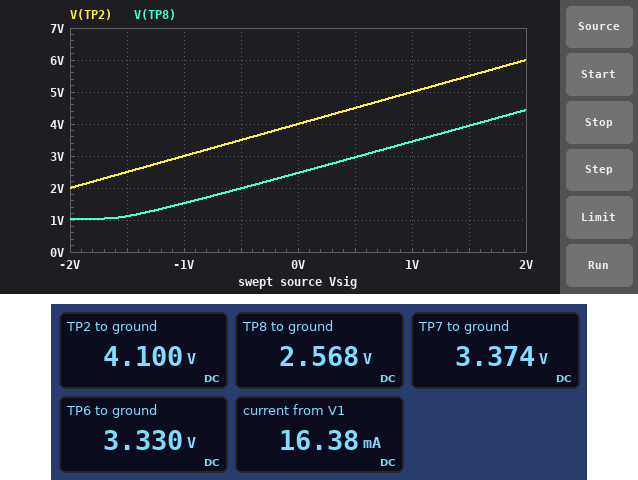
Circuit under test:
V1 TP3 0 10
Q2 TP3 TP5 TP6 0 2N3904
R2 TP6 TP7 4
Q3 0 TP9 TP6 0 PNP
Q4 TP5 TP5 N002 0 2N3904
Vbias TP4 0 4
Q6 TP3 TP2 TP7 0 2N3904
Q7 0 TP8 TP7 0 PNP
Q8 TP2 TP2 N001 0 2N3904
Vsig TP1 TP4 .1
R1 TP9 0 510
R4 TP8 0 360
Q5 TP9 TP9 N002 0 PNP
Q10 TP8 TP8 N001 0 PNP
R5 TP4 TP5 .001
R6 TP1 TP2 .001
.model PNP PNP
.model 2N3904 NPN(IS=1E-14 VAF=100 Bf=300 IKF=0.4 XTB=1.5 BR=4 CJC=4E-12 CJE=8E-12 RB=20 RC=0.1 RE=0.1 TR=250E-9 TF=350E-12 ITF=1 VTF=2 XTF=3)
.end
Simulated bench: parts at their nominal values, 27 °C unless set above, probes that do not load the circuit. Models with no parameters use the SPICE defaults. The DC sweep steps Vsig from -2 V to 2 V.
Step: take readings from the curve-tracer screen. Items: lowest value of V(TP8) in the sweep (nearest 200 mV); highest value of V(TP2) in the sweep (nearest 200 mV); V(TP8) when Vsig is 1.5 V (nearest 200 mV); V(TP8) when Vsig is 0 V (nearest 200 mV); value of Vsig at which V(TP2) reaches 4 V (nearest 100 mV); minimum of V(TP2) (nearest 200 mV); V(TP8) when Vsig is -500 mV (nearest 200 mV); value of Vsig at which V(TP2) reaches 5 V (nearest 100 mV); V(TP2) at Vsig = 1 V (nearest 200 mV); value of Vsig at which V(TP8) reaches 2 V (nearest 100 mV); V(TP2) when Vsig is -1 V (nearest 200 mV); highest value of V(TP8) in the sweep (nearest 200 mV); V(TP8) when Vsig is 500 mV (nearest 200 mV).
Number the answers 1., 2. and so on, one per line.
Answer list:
1. 1.0 V
2. 6.0 V
3. 4.0 V
4. 2.4 V
5. 0 V
6. 2.0 V
7. 2.0 V
8. 1.0 V
9. 5.0 V
10. -500 mV
11. 3.0 V
12. 4.4 V
13. 3.0 V
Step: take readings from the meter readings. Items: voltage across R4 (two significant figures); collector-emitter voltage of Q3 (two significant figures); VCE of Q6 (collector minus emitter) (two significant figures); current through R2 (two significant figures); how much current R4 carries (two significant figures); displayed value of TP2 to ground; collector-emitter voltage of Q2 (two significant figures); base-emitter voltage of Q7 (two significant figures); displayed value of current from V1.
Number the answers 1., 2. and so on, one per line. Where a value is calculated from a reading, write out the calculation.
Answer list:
1. 2.568 V = 2.6 V
2. 0 V - 3.33 V = -3.3 V
3. 10 V - 3.374 V = 6.6 V
4. (3.374 V - 3.33 V) / 4 Ω = 11 mA
5. (2.568 V) / 360 Ω = 7.1 mA
6. 4.100 V
7. 10 V - 3.33 V = 6.7 V
8. 2.568 V - 3.374 V = -810 mV
9. 16.38 mA
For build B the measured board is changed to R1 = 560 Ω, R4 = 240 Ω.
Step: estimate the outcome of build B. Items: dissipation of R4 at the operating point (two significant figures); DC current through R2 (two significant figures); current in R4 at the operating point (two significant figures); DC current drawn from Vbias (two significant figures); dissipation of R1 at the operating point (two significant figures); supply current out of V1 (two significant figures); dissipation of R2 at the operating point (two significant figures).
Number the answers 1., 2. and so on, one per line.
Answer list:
1. 27 mW
2. 9.7 mA
3. 11 mA
4. 15 mA
5. 11 mW
6. 18 mA
7. 380 µW
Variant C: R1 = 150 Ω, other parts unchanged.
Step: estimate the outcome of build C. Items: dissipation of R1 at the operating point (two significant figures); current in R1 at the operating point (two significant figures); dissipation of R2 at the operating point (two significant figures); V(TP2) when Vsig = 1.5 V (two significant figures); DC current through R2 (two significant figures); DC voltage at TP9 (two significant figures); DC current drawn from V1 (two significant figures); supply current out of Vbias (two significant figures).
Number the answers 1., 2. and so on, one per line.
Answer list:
1. 39 mW
2. 16 mA
3. 1.5 mW
4. 5.5 V
5. 19 mA
6. 2.4 V
7. 31 mA
8. 23 mA
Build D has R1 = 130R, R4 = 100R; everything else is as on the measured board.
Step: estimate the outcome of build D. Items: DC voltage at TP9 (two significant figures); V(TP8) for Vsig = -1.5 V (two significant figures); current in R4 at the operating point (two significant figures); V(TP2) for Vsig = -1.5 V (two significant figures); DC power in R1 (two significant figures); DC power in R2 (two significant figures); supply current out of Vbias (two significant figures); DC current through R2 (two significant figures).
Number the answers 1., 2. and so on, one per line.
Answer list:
1. 2.4 V
2. 970 mV
3. 25 mA
4. 2.5 V
5. 45 mW
6. 1.2 mW
7. 43 mA
8. 17 mA
